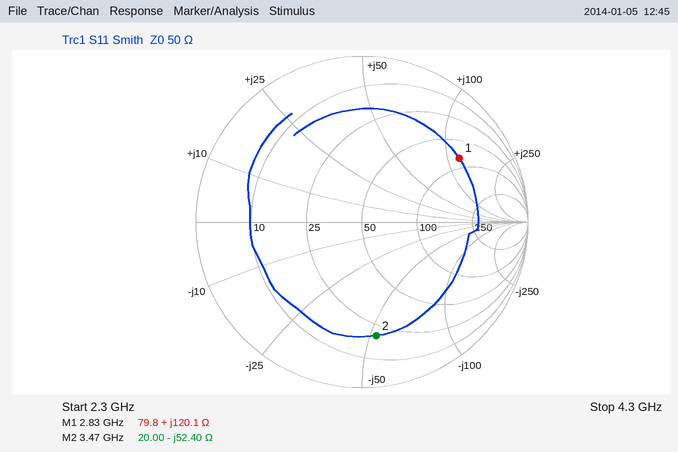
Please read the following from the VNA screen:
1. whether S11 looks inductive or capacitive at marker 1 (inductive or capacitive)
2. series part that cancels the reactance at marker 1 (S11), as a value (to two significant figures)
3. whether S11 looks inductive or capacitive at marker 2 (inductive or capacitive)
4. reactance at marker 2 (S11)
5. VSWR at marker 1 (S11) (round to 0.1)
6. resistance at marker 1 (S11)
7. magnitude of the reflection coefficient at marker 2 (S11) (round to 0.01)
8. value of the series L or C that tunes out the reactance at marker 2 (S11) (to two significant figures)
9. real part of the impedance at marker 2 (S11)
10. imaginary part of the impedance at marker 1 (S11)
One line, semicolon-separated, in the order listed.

inductive; 470 fF; capacitive; -52.40 Ω; 5.7; 79.8 Ω; 0.69; 2.4 nH; 20.00 Ω; +120.1 Ω
